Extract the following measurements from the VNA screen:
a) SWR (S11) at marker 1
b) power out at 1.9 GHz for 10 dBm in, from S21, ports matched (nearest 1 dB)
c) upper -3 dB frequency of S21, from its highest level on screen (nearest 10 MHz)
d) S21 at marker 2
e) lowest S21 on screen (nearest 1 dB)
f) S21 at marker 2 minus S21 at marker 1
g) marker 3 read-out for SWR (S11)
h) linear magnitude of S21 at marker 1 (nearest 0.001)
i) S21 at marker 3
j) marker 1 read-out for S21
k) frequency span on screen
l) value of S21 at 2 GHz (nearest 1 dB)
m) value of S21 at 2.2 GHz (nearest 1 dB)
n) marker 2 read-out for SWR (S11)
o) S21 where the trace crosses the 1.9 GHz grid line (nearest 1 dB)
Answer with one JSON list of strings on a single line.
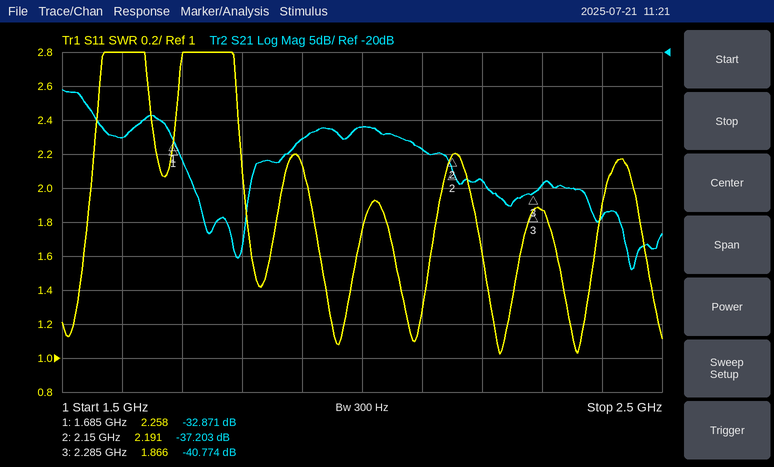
["2.258", "-23 dBm", "1.55 GHz", "-37.203 dB", "-52 dB", "-4.332 dB", "1.866", "0.023", "-40.774 dB", "-32.871 dB", "1 GHz", "-31 dB", "-39 dB", "2.191", "-33 dB"]
